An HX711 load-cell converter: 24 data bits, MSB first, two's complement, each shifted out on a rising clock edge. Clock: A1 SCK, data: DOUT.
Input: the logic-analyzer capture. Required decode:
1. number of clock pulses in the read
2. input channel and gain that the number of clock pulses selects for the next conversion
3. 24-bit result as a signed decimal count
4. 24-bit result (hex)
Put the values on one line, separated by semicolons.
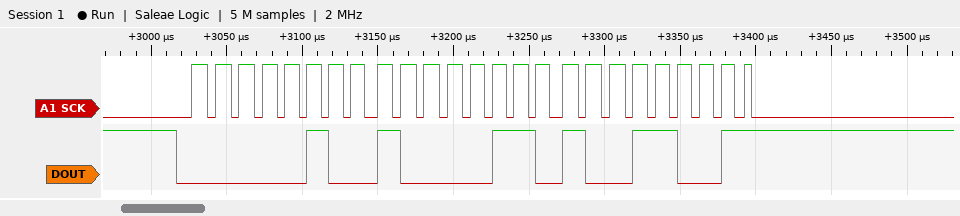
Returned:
25; channel A, gain 128; 296601; 0x048699
